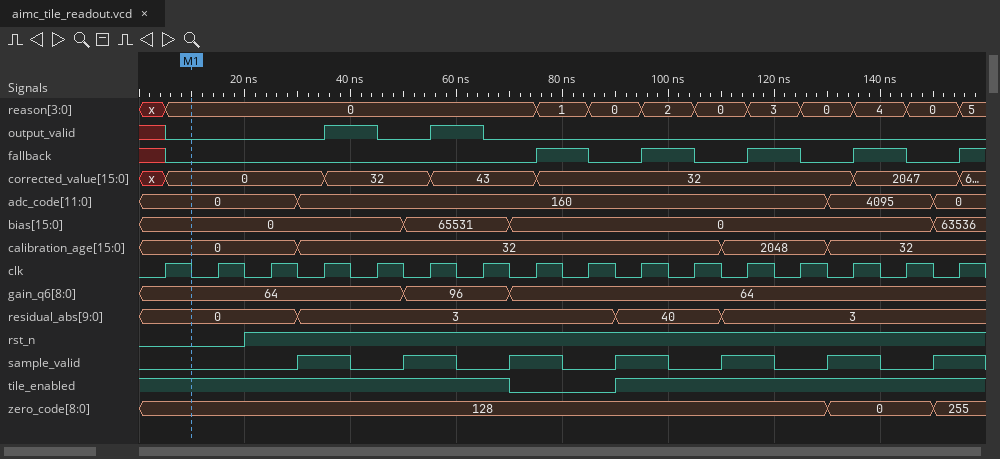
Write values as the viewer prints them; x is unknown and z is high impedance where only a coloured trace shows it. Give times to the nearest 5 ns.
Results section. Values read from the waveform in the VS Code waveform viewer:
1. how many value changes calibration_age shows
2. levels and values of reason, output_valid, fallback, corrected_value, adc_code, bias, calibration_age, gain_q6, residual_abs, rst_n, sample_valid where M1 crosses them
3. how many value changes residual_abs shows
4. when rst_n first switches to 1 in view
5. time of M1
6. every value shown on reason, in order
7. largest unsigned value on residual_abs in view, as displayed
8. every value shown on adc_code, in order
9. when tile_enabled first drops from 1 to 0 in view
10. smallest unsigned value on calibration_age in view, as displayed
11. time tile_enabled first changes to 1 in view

3
reason=0, output_valid=0, fallback=0, corrected_value=0, adc_code=0, bias=0, calibration_age=0, gain_q6=64, residual_abs=0, rst_n=0, sample_valid=0
3
20 ns
10 ns
x, 0, 1, 0, 2, 0, 3, 0, 4, 0, 5
40
0, 160, 4095, 0
70 ns
0
90 ns
